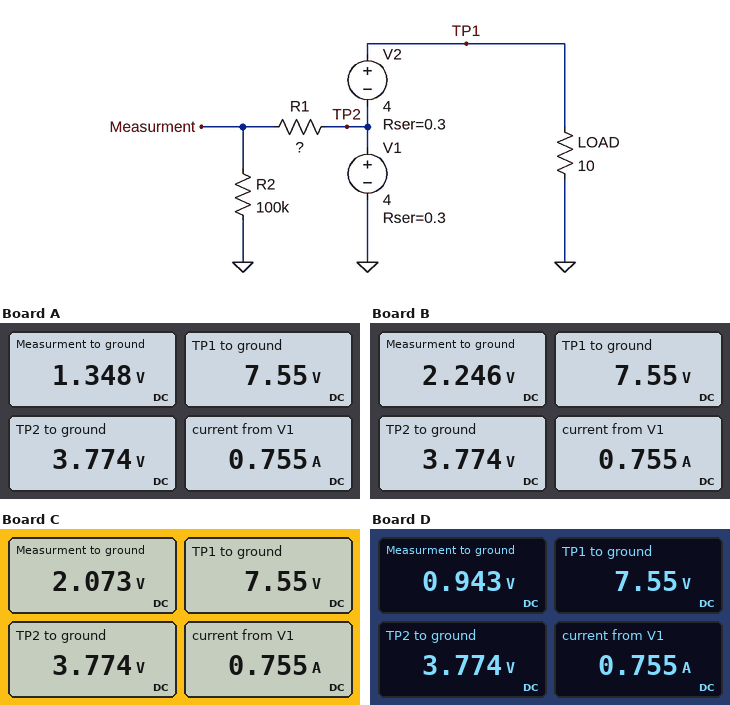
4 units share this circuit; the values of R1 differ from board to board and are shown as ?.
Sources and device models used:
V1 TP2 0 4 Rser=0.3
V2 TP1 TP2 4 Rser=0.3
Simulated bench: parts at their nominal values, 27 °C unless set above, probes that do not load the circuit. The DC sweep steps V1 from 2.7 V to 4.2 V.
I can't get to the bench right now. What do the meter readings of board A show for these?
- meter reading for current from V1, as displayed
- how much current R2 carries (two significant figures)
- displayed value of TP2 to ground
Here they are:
0.755 A
13 µA
3.774 V
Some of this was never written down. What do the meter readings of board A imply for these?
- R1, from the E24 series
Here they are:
180 kΩ
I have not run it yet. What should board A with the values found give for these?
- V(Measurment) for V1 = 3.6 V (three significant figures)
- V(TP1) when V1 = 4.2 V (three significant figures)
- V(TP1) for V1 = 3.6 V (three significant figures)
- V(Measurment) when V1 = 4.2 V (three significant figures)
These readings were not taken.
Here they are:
1.21 V
7.74 V
7.17 V
1.42 V
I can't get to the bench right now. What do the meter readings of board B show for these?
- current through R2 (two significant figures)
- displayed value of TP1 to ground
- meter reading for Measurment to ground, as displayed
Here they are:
22 µA
7.55 V
2.246 V
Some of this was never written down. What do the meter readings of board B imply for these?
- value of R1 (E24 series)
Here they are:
68 kΩ
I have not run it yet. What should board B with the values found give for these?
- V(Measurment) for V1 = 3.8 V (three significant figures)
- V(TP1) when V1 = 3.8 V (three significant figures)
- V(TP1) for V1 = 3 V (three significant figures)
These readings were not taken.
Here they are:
2.13 V
7.36 V
6.60 V
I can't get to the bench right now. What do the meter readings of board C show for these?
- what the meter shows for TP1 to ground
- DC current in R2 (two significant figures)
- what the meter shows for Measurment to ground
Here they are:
7.55 V
21 µA
2.073 V
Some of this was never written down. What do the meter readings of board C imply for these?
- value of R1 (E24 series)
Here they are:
82 kΩ
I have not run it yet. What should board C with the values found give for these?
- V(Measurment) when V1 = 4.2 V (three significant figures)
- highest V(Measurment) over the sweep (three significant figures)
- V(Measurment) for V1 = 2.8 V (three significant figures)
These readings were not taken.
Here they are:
2.18 V
2.18 V
1.43 V
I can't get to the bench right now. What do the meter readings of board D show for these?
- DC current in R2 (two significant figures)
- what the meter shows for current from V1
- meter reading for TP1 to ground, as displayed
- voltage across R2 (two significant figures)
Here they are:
9.4 µA
0.755 A
7.55 V
940 mV
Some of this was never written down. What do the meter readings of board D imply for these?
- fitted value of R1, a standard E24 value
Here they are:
300 kΩ
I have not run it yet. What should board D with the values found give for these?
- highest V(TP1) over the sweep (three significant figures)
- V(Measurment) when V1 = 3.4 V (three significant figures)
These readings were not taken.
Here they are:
7.74 V
798 mV
